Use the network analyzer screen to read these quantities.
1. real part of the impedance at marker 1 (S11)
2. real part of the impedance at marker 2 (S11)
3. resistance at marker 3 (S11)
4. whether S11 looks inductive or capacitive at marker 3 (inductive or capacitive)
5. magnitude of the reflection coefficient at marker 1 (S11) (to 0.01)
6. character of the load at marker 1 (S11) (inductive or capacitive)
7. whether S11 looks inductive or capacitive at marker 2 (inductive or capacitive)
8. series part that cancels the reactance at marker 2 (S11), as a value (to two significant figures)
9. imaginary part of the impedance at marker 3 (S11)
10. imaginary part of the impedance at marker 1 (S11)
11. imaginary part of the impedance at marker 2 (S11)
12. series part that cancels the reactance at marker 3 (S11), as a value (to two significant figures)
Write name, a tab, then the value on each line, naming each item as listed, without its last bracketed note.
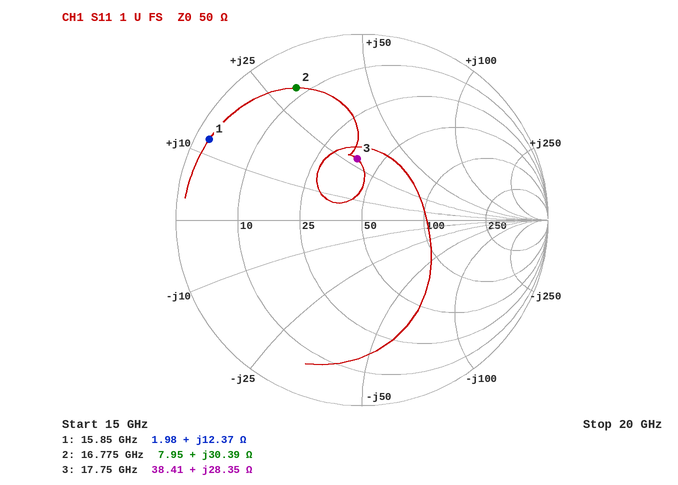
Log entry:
real part of the impedance at marker 1	1.98 Ω
real part of the impedance at marker 2	7.95 Ω
resistance at marker 3	38.41 Ω
whether S11 looks inductive or capacitive at marker 3	inductive
magnitude of the reflection coefficient at marker 1 (S11)	0.93
character of the load at marker 1 (S11)	inductive
whether S11 looks inductive or capacitive at marker 2	inductive
series part that cancels the reactance at marker 2 (S11), as a value	310 fF
imaginary part of the impedance at marker 3	+28.35 Ω
imaginary part of the impedance at marker 1	+12.37 Ω
imaginary part of the impedance at marker 2	+30.39 Ω
series part that cancels the reactance at marker 3 (S11), as a value	320 fF
